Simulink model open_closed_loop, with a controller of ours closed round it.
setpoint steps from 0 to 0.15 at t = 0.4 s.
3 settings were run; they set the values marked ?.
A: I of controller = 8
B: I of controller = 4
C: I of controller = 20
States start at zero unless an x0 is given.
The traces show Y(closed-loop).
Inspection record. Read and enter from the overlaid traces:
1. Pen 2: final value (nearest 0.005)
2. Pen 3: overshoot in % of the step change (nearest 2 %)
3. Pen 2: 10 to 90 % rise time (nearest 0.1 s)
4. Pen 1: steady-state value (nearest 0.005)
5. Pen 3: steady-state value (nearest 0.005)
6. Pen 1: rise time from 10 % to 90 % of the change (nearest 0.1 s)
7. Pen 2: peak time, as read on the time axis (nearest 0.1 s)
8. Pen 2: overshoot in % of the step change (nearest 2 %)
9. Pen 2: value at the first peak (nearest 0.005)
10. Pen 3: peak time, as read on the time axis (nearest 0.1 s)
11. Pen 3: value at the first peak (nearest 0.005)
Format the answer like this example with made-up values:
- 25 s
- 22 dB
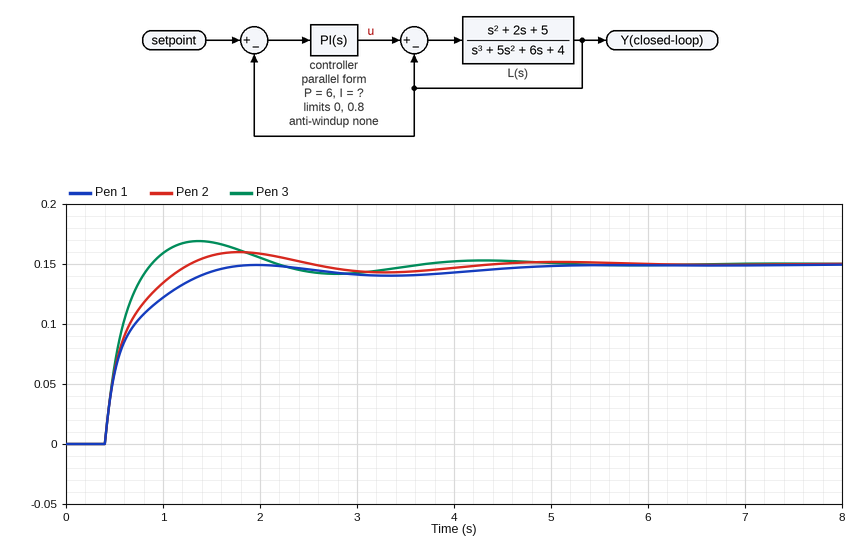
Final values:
- 0.150
- 12 %
- 0.6 s
- 0.150
- 0.150
- 0.8 s
- 1.8 s
- 6 %
- 0.160
- 1.4 s
- 0.170
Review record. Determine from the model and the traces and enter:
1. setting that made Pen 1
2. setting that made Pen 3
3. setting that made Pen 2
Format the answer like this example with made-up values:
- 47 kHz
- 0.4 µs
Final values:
- B
- C
- A
